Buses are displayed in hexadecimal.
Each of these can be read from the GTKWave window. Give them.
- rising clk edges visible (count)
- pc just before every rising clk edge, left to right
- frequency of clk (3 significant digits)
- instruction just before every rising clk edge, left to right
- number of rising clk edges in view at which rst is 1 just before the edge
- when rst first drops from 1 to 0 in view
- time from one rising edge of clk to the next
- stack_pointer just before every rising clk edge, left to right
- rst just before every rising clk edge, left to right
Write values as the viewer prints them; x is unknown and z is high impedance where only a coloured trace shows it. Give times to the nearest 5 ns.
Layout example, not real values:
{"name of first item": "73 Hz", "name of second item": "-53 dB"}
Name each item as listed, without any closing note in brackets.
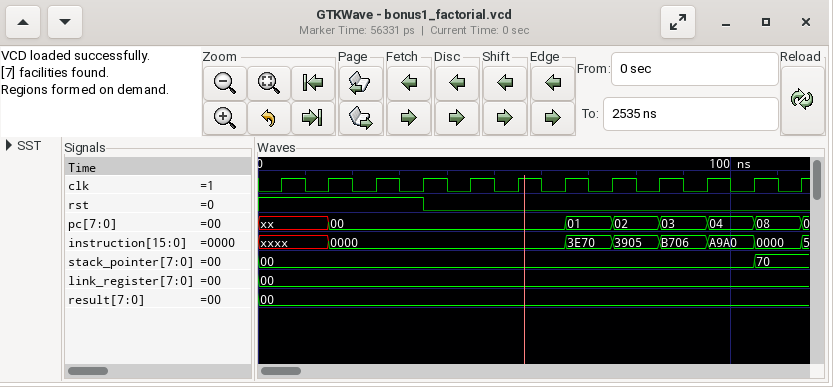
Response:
{"rising clk edges visible": "12", "pc just before every rising clk edge, left to right": "xx, xx, 00, 00, 00, 00, 00, 01, 02, 03, 04, 08", "frequency of clk": "100 MHz", "instruction just before every rising clk edge, left to right": "xxxx, xxxx, 0000, 0000, 0000, 0000, 0000, 3E70, 3905, B706, A9A0, 0000", "number of rising clk edges in view at which rst is 1 just before the edge": "4", "when rst first drops from 1 to 0 in view": "35 ns", "time from one rising edge of clk to the next": "10 ns", "stack_pointer just before every rising clk edge, left to right": "00, 00, 00, 00, 00, 00, 00, 00, 00, 00, 00, 70", "rst just before every rising clk edge, left to right": "1 1 1 1 0 0 0 0 0 0 0 0"}
